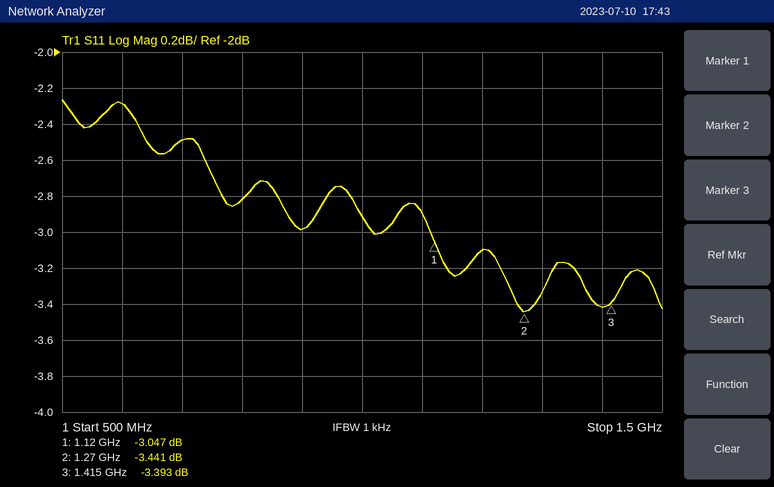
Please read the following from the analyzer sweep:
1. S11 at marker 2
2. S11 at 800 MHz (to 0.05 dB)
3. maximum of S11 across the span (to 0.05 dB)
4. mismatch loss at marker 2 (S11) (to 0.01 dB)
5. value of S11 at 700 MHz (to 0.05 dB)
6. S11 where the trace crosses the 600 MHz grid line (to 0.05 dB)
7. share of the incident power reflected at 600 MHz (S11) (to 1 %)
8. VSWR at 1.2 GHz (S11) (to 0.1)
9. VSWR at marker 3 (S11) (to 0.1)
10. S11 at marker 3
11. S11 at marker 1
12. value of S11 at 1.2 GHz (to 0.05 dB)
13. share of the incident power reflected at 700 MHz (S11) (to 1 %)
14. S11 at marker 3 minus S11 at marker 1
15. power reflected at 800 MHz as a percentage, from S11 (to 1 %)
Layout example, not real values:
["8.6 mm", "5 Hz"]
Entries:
["-3.441 dB", "-2.80 dB", "-2.25 dB", "2.62 dB", "-2.50 dB", "-2.30 dB", "59 %", "5.7", "5.2", "-3.393 dB", "-3.047 dB", "-3.10 dB", "56 %", "-0.346 dB", "52 %"]
